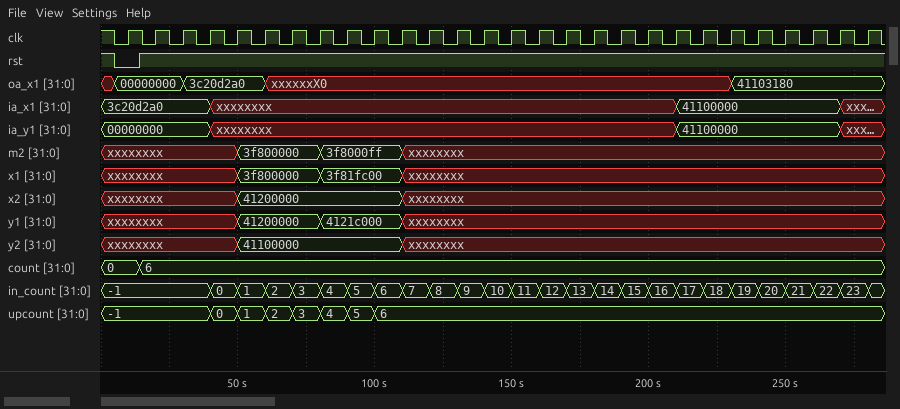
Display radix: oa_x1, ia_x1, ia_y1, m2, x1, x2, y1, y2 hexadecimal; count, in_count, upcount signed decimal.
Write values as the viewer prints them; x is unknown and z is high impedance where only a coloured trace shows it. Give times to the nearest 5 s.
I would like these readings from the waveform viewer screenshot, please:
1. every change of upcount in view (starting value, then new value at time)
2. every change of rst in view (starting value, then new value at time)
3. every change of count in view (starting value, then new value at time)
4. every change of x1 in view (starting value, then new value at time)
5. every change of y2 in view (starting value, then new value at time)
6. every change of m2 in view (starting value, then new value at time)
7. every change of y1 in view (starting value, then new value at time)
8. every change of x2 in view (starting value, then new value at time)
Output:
-1, 0 at 40 s, 1 at 50 s, 2 at 60 s, 3 at 70 s, 4 at 80 s, 5 at 90 s, 6 at 100 s
1, 0 at 5 s, 1 at 15 s
0, 6 at 15 s
xxxxxxxx, 3f800000 at 50 s, 3f81fc00 at 80 s, xxxxxxxx at 110 s
xxxxxxxx, 41100000 at 50 s, xxxxxxxx at 110 s
xxxxxxxx, 3f800000 at 50 s, 3f8000ff at 80 s, xxxxxxxx at 110 s
xxxxxxxx, 41200000 at 50 s, 4121c000 at 80 s, xxxxxxxx at 110 s
xxxxxxxx, 41200000 at 50 s, xxxxxxxx at 110 s
